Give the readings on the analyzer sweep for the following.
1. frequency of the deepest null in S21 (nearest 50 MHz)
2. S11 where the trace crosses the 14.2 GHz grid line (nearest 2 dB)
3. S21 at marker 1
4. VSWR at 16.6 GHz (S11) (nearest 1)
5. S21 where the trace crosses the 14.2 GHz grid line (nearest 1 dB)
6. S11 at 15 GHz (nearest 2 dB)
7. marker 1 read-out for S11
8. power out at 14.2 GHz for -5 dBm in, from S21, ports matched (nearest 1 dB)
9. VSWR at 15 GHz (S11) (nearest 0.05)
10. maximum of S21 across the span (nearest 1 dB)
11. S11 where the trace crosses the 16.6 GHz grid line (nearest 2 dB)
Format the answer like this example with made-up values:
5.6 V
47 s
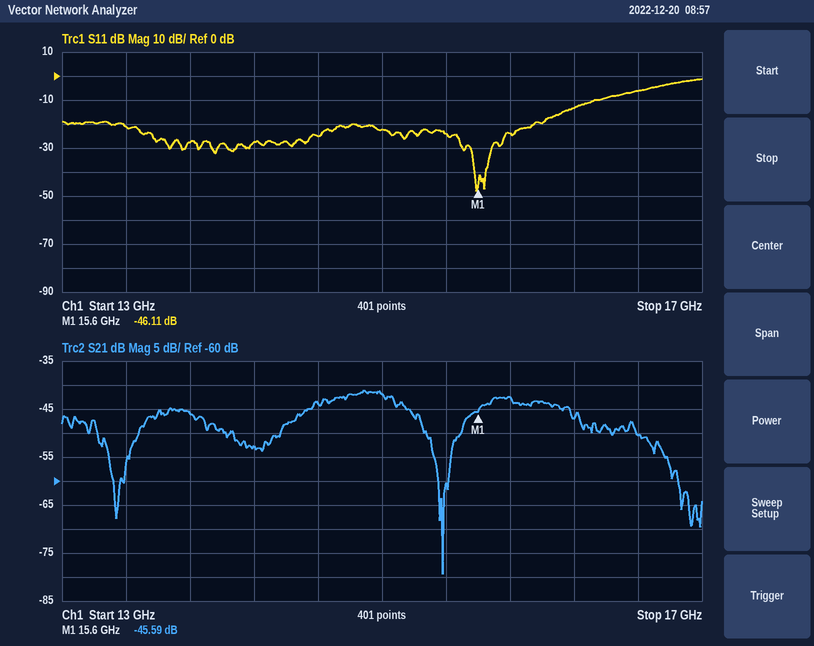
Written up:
15.40 GHz
-28 dB
-45.59 dB
3
-53 dB
-22 dB
-46.11 dB
-58 dBm
1.15
-41 dB
-6 dB
